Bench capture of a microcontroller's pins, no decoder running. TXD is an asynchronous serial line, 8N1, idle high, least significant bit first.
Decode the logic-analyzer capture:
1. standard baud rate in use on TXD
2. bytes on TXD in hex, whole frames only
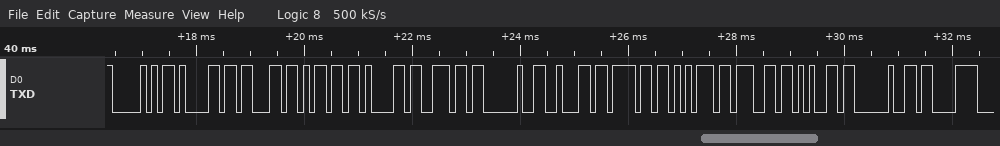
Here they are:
9600 baud
0x50 0x61 0x63 0x6D 0x61 0x6E 0x20 0x62 0x6F 0x75 0x67 0x65 0x20 0xC3
